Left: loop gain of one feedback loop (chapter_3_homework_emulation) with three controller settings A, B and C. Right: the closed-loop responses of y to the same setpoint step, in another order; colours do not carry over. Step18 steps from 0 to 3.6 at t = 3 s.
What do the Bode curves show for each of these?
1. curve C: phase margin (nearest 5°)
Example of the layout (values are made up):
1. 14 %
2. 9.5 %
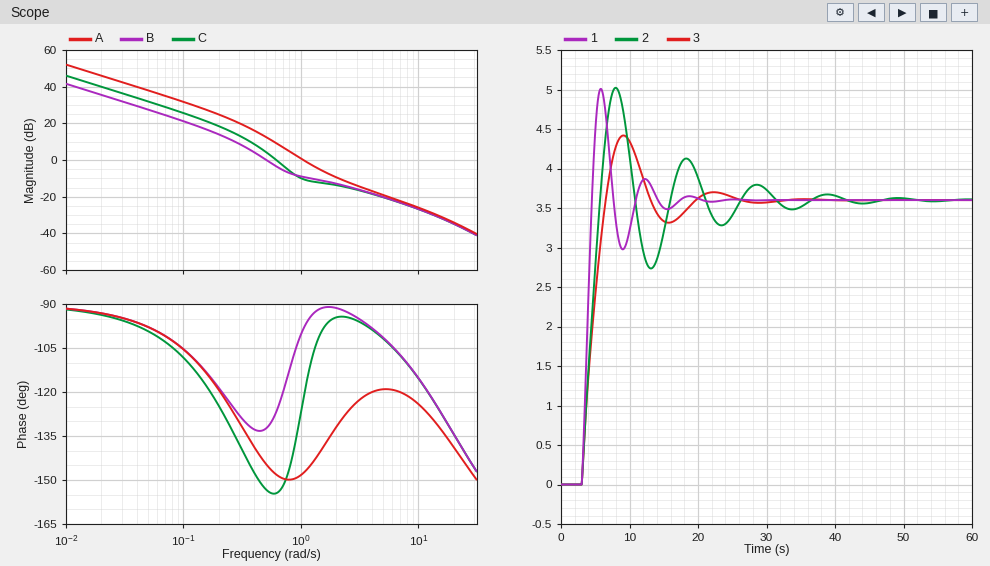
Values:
1. 25°
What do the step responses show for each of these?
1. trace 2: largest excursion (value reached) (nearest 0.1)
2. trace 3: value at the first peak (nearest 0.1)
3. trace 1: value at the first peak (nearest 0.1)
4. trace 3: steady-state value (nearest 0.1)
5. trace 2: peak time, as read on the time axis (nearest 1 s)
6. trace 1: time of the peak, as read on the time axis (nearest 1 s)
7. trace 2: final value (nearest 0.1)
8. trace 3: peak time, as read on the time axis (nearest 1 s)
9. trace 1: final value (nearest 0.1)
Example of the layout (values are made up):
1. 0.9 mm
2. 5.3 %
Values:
1. 5.0
2. 4.4
3. 5.0
4. 3.6
5. 8 s
6. 6 s
7. 3.6
8. 9 s
9. 3.6
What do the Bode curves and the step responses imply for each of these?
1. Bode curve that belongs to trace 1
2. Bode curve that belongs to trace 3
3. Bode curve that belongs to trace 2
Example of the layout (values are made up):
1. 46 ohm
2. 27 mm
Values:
1. A
2. B
3. C
